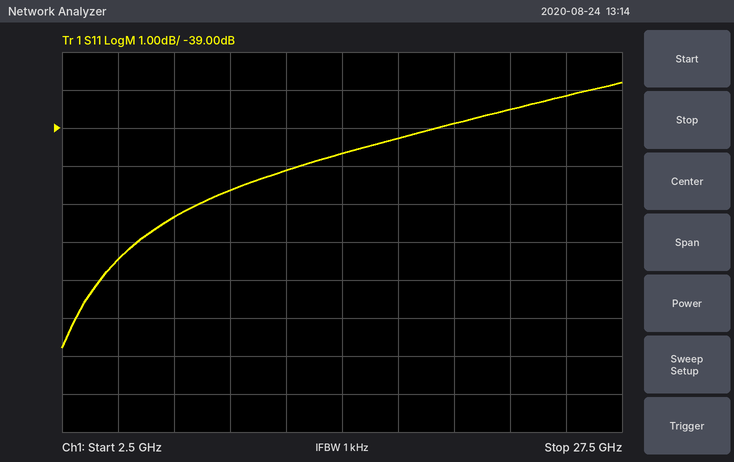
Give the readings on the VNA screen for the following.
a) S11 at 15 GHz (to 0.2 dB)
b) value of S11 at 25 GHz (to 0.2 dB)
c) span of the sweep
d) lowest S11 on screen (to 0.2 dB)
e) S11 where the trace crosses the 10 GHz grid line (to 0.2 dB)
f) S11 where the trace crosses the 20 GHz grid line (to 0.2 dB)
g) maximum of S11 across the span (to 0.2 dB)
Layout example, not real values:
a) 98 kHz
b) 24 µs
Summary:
a) -39.6 dB
b) -38.2 dB
c) 25 GHz
d) -44.8 dB
e) -40.6 dB
f) -38.8 dB
g) -37.8 dB
